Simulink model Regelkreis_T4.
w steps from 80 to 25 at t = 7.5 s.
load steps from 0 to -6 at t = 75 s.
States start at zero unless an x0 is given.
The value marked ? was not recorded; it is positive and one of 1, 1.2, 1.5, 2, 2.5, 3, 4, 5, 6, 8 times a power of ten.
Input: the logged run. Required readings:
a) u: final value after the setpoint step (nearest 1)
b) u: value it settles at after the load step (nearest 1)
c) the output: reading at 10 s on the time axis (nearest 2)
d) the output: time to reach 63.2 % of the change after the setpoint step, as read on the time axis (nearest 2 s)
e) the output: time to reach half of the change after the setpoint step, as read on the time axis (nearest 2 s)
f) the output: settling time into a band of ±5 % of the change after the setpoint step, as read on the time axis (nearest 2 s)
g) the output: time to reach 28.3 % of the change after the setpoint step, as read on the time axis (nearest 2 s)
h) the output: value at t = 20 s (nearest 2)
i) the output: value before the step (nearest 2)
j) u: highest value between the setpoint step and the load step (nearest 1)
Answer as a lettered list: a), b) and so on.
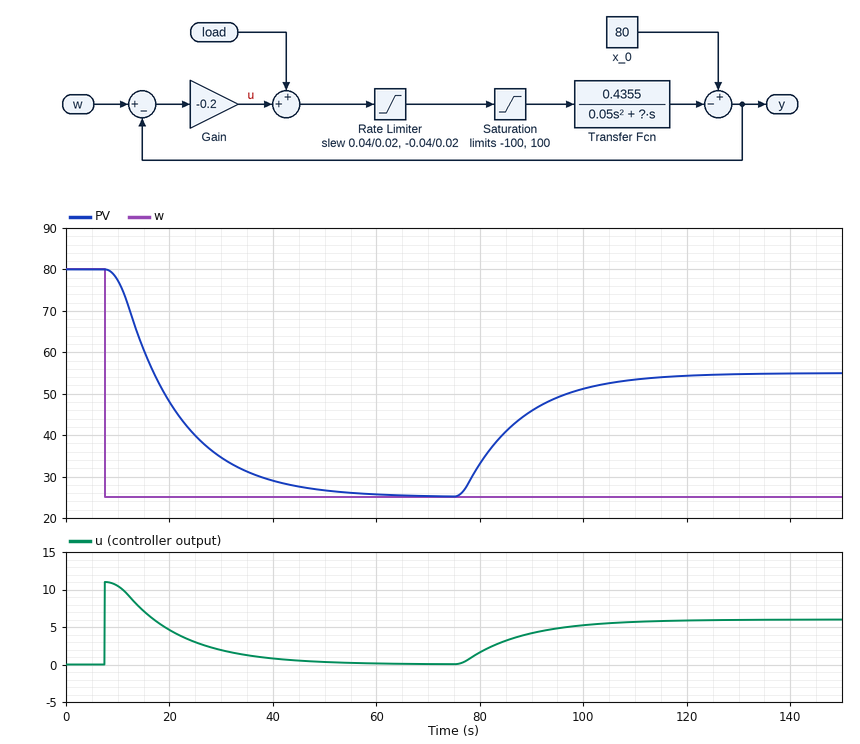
a) 0
b) 6
c) 78
d) 22 s
e) 18 s
f) 44 s
g) 14 s
h) 48
i) 80
j) 11
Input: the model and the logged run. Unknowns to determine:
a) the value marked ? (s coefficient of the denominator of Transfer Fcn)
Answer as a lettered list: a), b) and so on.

a) 1
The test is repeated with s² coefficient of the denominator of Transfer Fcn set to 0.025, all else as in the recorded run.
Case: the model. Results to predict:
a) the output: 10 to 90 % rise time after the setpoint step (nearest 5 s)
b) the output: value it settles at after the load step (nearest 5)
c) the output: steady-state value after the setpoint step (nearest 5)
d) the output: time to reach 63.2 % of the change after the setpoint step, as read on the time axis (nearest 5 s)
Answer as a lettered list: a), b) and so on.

a) 25 s
b) 55
c) 25
d) 20 s
